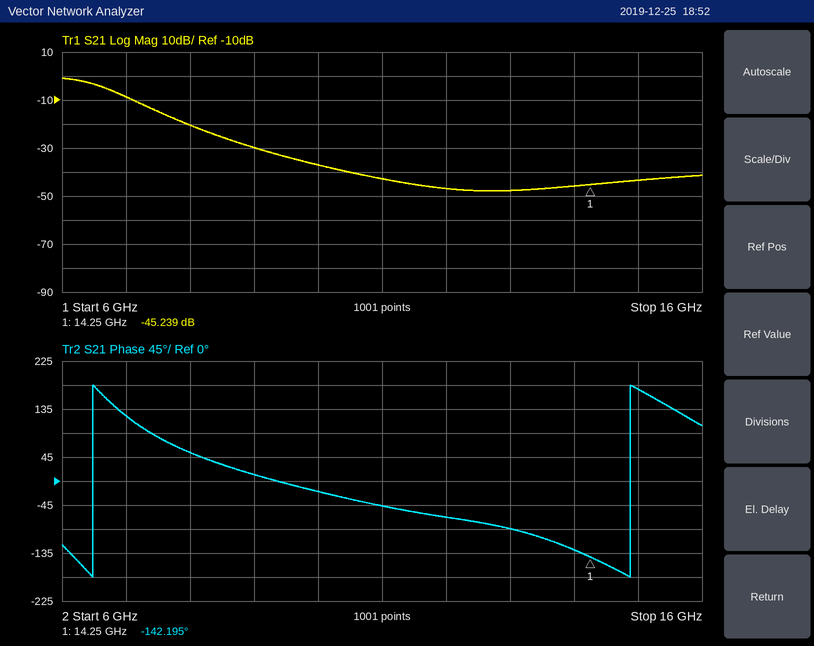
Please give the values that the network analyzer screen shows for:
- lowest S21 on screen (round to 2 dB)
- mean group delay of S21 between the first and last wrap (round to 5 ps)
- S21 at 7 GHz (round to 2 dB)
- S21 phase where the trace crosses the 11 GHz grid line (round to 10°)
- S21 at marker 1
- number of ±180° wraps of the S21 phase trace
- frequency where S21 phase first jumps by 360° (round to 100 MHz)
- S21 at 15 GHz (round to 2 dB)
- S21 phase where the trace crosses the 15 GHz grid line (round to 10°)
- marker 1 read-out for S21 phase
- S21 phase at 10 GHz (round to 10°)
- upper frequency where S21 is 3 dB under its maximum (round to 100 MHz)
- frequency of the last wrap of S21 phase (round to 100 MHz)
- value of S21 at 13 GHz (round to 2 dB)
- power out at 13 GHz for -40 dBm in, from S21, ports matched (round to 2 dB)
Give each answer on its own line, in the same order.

-48 dB
120 ps
-8 dB
-50°
-45.239 dB
2
6.5 GHz
-44 dB
170°
-142.195°
-20°
6.6 GHz
14.9 GHz
-48 dB
-88 dBm
